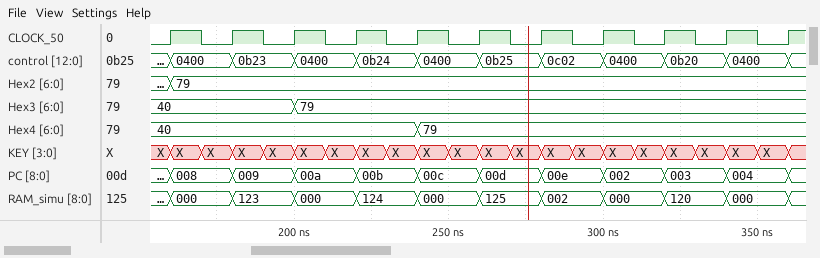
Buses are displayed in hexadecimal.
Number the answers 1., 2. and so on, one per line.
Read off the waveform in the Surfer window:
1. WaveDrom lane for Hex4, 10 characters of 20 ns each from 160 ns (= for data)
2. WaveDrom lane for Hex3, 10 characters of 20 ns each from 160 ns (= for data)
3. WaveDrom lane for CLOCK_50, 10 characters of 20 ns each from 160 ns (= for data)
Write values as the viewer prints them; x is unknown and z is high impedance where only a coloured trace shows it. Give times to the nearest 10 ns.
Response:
1. {name: 'Hex4', wave: '=...=.....', data: '40 79'}
2. {name: 'Hex3', wave: '=.=.......', data: '40 79'}
3. {name: 'CLOCK_50', wave: 'p.........'}
